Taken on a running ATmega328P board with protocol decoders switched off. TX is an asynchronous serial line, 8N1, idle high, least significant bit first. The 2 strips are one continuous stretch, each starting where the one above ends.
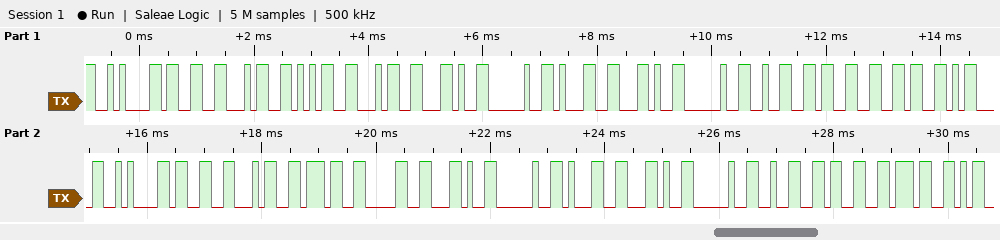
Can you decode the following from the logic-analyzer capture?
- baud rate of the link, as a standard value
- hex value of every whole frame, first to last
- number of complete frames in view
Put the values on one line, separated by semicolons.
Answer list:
9600 baud; 0A 33 34 35 34 2C 20 31 2C 20 32 33 36 0D 0A 33 34 37 30 2C 20 31 2C 20 32 33 37; 27
